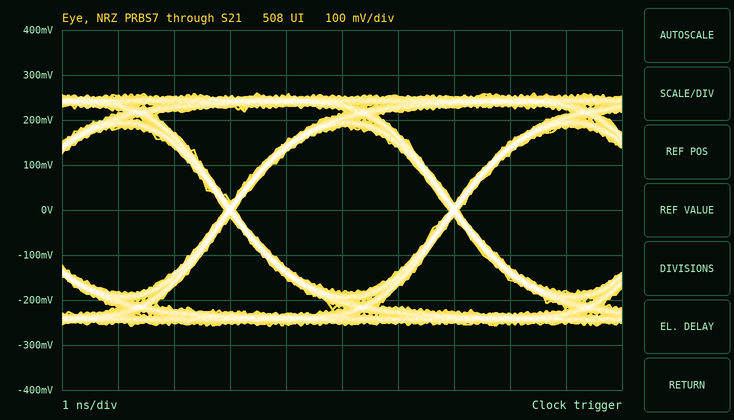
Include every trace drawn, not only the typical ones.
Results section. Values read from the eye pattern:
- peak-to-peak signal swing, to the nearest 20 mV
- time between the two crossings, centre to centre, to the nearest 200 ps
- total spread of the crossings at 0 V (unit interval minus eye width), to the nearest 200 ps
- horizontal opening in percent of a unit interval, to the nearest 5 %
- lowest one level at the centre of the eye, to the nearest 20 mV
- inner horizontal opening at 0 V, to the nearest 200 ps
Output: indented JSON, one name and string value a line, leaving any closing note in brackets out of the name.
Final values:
{
  "peak-to-peak signal swing, to the nearest 20 mV": "520 mV",
  "time between the two crossings, centre to centre, to the nearest 200 ps": "4.0 ns",
  "total spread of the crossings at 0 V (unit interval minus eye width), to the nearest 200 ps": "200 ps",
  "horizontal opening in percent of a unit interval, to the nearest 5 %": "95 %",
  "lowest one level at the centre of the eye, to the nearest 20 mV": "180 mV",
  "inner horizontal opening at 0 V, to the nearest 200 ps": "3.8 ns"
}
